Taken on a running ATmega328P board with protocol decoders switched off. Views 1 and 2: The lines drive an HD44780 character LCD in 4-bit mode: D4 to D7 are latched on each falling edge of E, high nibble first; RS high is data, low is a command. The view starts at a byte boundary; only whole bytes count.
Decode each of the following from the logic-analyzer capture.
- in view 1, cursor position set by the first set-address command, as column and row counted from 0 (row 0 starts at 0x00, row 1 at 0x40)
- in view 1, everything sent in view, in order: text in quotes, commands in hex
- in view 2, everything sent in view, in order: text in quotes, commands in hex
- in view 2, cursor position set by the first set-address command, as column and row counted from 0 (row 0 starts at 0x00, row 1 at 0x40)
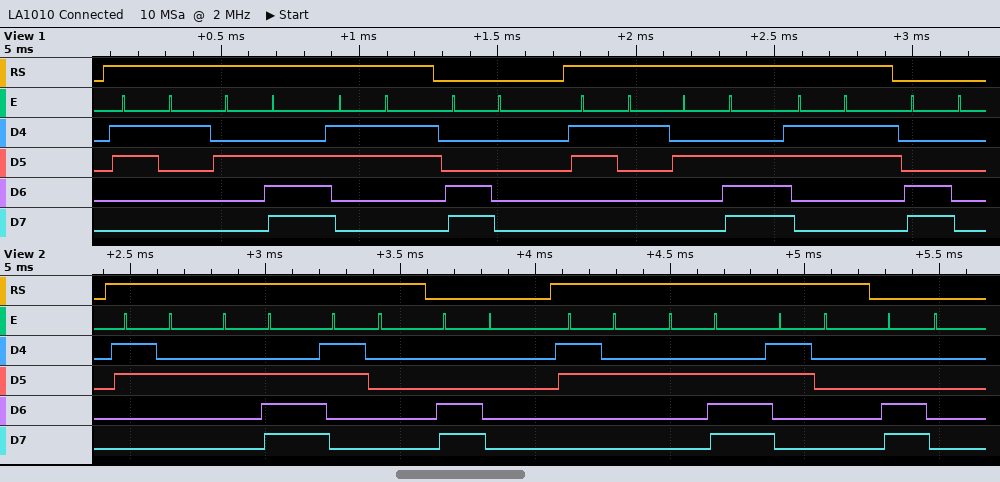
column 0, row 1
"1.3" 0xC0 "1.3" 0xC0
"2.0" 0xC0 "2.0" 0xC0
column 0, row 1
